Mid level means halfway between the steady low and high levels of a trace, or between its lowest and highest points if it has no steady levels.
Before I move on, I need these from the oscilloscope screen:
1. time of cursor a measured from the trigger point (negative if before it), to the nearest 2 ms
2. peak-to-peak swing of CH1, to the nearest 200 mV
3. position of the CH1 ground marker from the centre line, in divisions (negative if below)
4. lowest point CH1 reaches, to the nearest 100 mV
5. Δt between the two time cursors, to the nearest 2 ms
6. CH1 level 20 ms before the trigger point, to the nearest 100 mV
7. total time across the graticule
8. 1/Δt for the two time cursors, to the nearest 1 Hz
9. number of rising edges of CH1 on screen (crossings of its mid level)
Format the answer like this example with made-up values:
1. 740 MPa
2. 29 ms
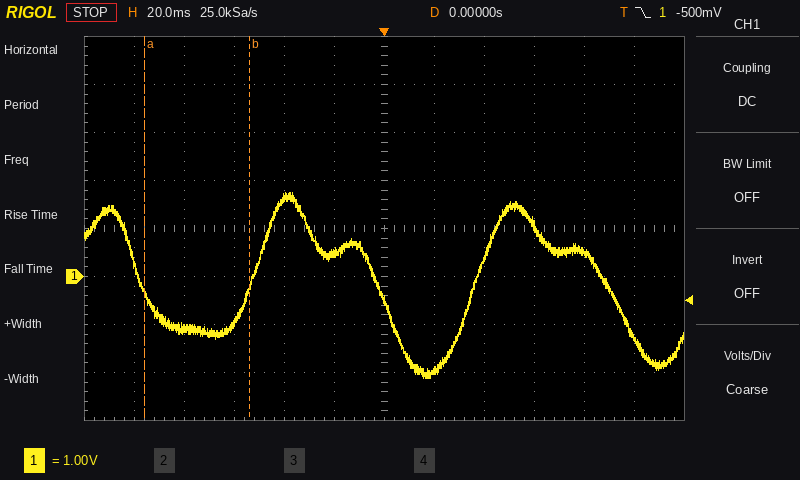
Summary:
1. -96 ms
2. 3.8 V
3. -1.0 div
4. -2.1 V
5. 42 ms
6. 500 mV
7. 240 ms
8. 24 Hz
9. 2
